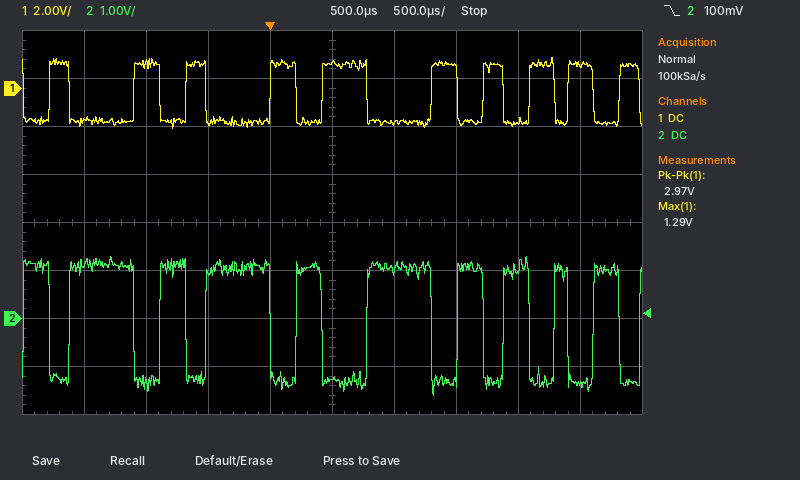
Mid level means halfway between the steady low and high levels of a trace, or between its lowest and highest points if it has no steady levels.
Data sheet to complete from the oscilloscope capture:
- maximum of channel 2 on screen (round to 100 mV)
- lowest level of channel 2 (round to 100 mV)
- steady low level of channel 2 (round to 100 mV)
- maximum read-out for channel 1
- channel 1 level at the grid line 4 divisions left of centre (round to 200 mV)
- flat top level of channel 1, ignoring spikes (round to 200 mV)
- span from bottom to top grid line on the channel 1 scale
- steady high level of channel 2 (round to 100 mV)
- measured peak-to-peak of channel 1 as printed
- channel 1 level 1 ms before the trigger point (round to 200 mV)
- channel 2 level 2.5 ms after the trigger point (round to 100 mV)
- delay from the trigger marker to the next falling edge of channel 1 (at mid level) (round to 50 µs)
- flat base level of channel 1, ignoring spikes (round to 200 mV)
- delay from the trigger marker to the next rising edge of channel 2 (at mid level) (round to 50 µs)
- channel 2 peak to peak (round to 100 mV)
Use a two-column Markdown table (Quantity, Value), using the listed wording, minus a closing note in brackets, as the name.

| Quantity | Value |
|---|---|
| maximum of channel 2 on screen | 1.3 V |
| lowest level of channel 2 | -1.6 V |
| steady low level of channel 2 | -1.3 V |
| maximum read-out for channel 1 | 1.29 V |
| channel 1 level at the grid line 4 divisions left of centre | -1.4 V |
| flat top level of channel 1, ignoring spikes | 1.0 V |
| span from bottom to top grid line on the channel 1 scale | 16 V |
| steady high level of channel 2 | 1.1 V |
| measured peak-to-peak of channel 1 as printed | 2.97 V |
| channel 1 level 1 ms before the trigger point | 1.0 V |
| channel 2 level 2.5 ms after the trigger point | -1.4 V |
| delay from the trigger marker to the next falling edge of channel 1 (at mid level) | 200 µs |
| flat base level of channel 1, ignoring spikes | -1.4 V |
| delay from the trigger marker to the next rising edge of channel 2 (at mid level) | 200 µs |
| channel 2 peak to peak | 2.9 V |
